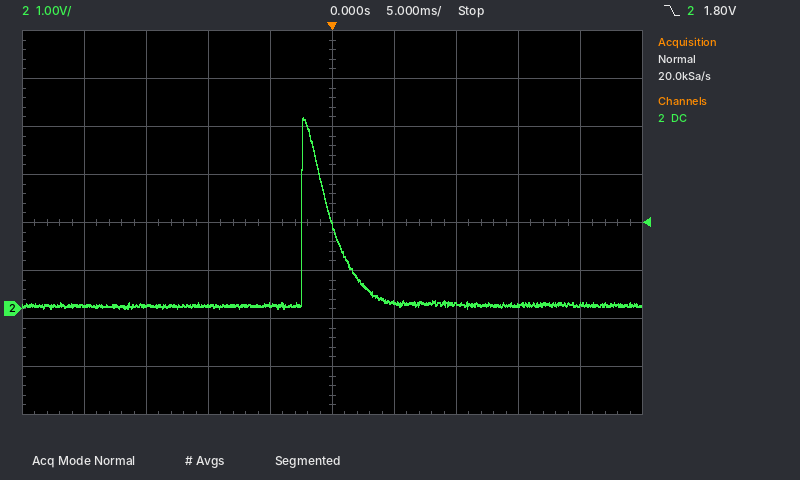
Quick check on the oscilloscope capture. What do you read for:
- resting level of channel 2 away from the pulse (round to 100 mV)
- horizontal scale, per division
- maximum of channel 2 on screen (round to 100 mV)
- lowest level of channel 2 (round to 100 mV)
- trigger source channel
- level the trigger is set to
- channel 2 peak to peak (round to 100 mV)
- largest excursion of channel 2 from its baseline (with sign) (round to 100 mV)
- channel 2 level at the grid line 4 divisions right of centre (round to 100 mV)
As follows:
100 mV
5 ms
4.0 V
0.0 V
channel 2
1.80 V
4.0 V
+3.9 V
100 mV
